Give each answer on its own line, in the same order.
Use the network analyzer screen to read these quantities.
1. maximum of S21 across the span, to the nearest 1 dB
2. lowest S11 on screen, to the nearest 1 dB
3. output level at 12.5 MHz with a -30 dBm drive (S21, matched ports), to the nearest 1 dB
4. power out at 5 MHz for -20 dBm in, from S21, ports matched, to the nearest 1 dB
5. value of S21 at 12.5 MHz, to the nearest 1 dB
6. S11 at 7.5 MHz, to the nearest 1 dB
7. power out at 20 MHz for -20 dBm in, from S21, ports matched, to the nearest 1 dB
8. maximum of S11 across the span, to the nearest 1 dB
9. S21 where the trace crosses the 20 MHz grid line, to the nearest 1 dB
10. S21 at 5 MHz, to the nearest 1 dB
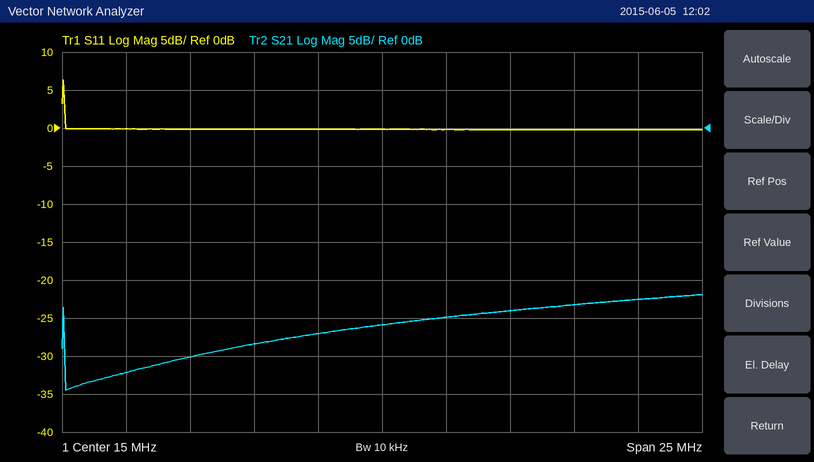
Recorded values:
-22 dB
0 dB
-57 dBm
-52 dBm
-27 dB
0 dB
-44 dBm
6 dB
-24 dB
-32 dB
